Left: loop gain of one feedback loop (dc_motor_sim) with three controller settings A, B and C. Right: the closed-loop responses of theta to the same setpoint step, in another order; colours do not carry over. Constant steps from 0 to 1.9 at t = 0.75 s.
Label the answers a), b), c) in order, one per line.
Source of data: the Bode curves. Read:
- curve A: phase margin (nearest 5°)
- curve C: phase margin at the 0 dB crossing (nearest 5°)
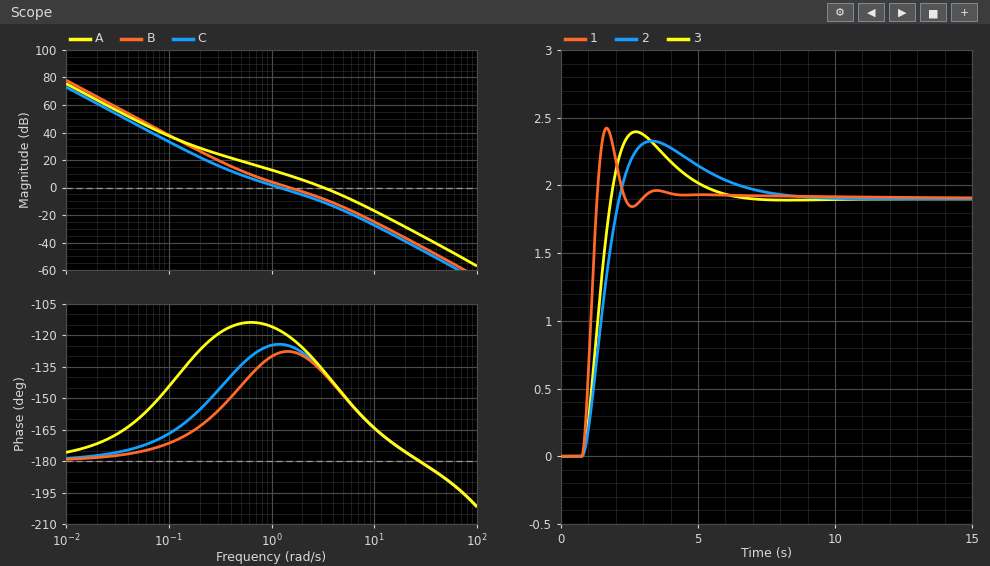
a) 45°
b) 55°
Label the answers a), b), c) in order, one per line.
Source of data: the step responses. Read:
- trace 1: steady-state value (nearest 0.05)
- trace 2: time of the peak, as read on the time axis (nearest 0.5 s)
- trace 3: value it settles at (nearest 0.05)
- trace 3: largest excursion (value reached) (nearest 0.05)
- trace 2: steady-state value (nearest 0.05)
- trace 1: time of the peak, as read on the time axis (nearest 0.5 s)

a) 1.90
b) 3.5 s
c) 1.90
d) 2.40
e) 1.90
f) 1.5 s
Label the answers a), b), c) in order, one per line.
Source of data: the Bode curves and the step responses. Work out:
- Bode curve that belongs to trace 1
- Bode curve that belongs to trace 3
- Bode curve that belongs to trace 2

a) A
b) B
c) C
